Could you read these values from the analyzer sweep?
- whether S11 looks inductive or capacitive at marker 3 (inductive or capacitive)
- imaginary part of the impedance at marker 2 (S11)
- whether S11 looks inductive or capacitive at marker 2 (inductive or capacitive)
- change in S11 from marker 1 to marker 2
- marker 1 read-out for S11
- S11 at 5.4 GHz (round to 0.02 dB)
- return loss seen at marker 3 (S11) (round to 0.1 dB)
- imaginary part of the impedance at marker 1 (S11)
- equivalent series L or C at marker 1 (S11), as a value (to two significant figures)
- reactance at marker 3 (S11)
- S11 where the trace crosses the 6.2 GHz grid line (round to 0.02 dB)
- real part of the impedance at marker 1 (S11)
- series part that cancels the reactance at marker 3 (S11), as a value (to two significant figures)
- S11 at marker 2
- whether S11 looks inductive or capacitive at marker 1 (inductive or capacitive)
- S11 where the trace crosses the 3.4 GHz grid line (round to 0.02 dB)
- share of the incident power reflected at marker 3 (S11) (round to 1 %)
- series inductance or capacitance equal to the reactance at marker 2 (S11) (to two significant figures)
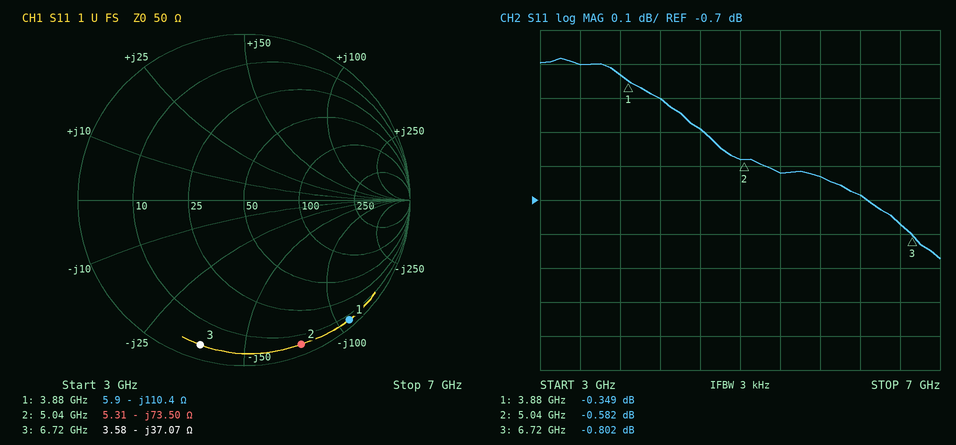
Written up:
capacitive
-73.50 Ω
capacitive
-0.233 dB
-0.349 dB
-0.62 dB
0.8 dB
-110.4 Ω
370 fF
-37.07 Ω
-0.68 dB
5.9 Ω
880 pH
-0.582 dB
capacitive
-0.30 dB
83 %
430 fF
